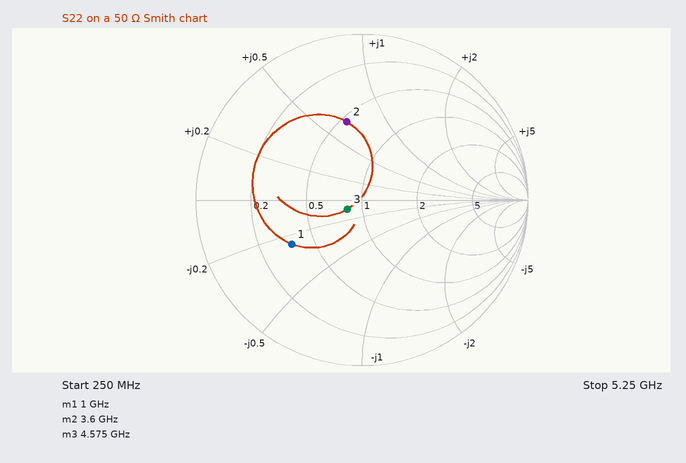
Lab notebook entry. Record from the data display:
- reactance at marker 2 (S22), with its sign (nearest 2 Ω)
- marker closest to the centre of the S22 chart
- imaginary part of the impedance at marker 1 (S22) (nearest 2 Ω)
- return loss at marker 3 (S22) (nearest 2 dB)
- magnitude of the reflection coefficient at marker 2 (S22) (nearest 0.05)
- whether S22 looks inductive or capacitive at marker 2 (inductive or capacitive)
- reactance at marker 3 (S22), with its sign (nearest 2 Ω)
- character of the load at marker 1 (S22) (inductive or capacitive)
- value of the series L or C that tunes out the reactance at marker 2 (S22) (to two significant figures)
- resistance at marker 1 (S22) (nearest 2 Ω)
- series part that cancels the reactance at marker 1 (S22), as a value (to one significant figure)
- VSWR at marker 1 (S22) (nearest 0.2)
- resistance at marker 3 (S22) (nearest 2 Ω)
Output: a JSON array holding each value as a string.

["+34 Ω", "marker 3", "-12 Ω", "20 dB", "0.50", "inductive", "-4 Ω", "capacitive", "1.3 pF", "18 Ω", "2 nH", "3.0", "42 Ω"]
